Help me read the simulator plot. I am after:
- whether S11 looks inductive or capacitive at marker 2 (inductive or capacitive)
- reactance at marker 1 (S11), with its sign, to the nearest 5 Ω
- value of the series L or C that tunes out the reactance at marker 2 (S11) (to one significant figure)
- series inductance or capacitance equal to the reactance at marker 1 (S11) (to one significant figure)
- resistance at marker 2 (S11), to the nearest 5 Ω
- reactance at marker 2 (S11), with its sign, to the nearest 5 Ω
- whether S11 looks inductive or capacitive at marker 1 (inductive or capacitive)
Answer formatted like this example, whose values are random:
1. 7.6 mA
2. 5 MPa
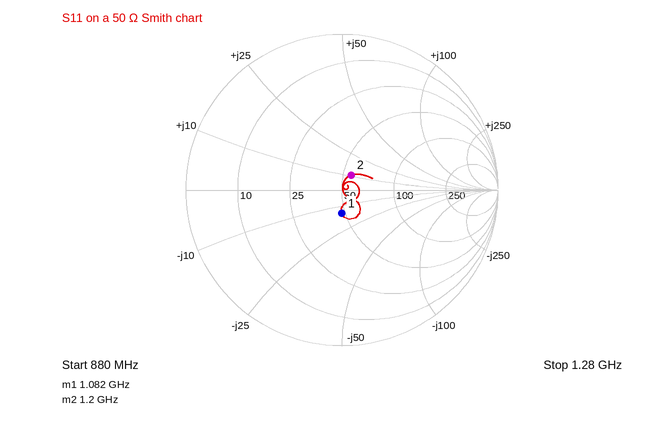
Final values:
1. inductive
2. -15 Ω
3. 10 pF
4. 10 pF
5. 55 Ω
6. +10 Ω
7. capacitive
